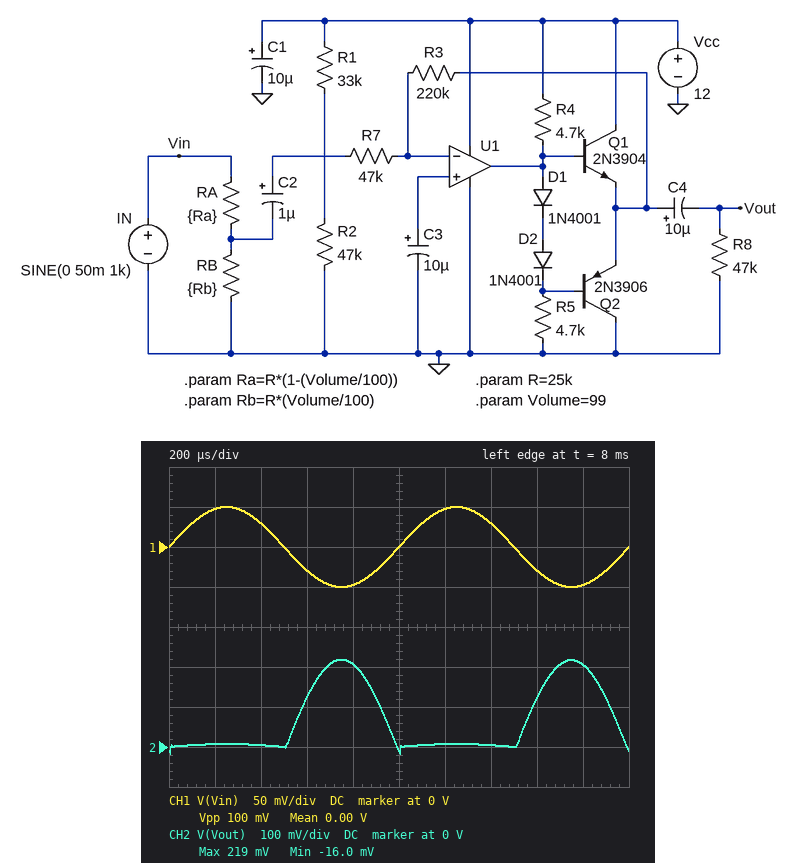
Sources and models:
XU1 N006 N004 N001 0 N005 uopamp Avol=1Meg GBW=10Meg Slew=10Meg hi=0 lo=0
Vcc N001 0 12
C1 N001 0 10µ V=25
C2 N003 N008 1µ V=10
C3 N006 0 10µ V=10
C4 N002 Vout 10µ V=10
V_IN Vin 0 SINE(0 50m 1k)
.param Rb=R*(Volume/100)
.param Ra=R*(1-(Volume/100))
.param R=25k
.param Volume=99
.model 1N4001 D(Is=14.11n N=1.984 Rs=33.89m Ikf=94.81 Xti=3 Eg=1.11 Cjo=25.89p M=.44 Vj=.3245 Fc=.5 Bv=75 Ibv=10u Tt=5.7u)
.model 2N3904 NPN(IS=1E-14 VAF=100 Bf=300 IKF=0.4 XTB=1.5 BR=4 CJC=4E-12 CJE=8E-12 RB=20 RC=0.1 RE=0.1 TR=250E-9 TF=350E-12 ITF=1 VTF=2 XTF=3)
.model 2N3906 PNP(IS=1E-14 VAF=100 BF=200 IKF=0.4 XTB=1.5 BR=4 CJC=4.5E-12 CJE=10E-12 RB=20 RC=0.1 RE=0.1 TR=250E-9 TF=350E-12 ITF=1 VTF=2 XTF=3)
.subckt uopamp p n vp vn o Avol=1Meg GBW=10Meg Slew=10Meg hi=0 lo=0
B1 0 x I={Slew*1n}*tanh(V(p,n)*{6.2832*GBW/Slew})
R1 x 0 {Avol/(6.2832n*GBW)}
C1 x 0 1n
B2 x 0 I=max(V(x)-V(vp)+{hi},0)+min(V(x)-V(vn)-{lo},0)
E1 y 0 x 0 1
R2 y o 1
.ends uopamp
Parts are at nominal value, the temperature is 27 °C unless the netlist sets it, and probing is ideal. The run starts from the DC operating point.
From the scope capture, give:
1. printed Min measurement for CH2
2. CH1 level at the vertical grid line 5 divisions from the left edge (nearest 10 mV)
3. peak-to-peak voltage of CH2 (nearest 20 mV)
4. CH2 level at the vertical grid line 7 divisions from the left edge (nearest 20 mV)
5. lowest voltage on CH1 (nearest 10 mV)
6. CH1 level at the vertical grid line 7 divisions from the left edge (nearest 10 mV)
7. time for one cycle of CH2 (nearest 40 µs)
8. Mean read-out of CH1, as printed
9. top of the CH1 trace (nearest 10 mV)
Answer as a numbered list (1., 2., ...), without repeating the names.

1. -16.0 mV
2. 0 V
3. 240 mV
4. 0 V
5. -50 mV
6. 30 mV
7. 1.00 ms
8. 0.00 V
9. 50 mV
